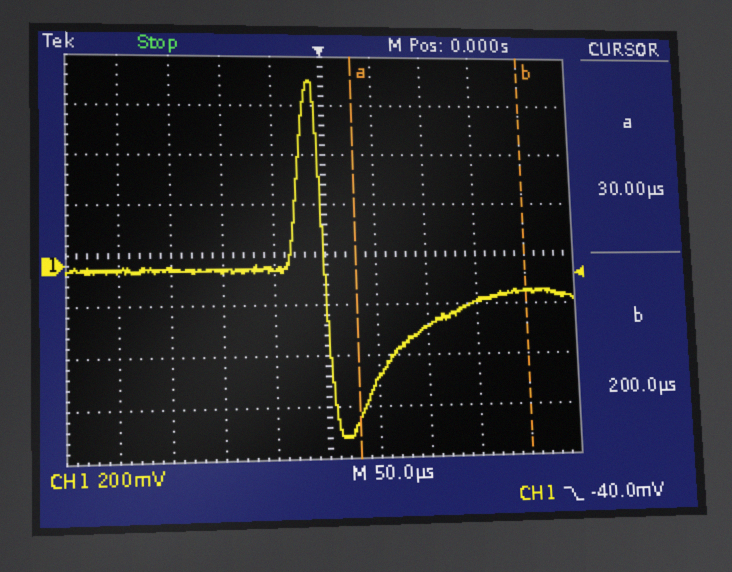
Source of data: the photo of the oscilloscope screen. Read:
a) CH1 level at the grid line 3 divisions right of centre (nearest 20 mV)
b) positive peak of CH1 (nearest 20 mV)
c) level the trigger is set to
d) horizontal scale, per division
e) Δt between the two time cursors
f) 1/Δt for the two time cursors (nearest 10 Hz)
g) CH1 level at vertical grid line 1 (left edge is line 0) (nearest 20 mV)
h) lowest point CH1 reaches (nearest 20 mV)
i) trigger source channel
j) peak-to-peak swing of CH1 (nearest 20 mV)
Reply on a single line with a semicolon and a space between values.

-140 mV; 740 mV; -40.0 mV; 50 µs; 170 µs; 5.88 kHz; -20 mV; -680 mV; CH1; 1.42 V
